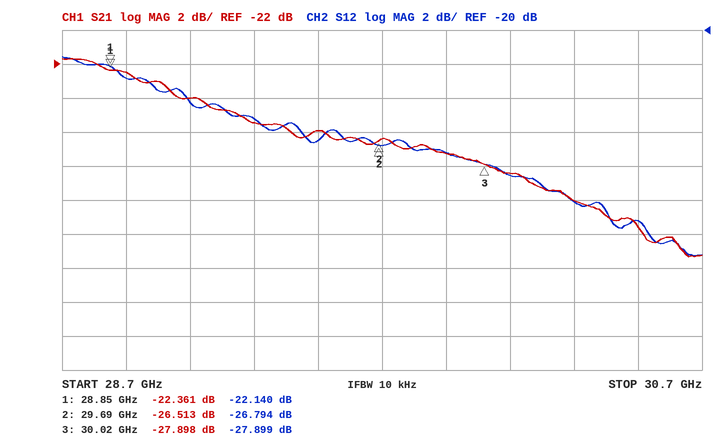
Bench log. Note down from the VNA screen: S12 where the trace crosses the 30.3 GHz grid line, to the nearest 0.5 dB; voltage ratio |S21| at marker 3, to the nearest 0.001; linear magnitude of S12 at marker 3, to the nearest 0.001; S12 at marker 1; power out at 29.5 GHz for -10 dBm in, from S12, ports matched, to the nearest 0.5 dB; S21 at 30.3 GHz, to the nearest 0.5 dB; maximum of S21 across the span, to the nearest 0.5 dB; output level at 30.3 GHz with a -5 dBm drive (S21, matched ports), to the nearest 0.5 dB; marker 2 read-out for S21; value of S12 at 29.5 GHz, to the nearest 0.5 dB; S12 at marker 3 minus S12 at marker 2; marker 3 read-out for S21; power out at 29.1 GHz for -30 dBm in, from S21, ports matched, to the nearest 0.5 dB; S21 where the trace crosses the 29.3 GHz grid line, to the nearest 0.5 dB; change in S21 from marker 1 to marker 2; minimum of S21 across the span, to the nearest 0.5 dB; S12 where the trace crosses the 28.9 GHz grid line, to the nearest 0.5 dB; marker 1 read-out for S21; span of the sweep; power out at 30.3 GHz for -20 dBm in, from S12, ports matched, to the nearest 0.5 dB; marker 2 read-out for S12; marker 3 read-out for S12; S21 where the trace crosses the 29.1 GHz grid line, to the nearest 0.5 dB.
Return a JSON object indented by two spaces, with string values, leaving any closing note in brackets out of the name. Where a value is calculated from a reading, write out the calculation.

{
  "S12 where the trace crosses the 30.3 GHz grid line, to the nearest 0.5 dB": "-30.0 dB",
  "voltage ratio |S21| at marker 3, to the nearest 0.001": "10^(-27.898/20) ≈ 0.040",
  "linear magnitude of S12 at marker 3, to the nearest 0.001": "10^(-27.899/20) ≈ 0.040",
  "S12 at marker 1": "-22.140 dB",
  "power out at 29.5 GHz for -10 dBm in, from S12, ports matched, to the nearest 0.5 dB": "-10 dBm + (-26.5 dB) = -36.5 dBm",
  "S21 at 30.3 GHz, to the nearest 0.5 dB": "-30.0 dB",
  "maximum of S21 across the span, to the nearest 0.5 dB": "-21.5 dB",
  "output level at 30.3 GHz with a -5 dBm drive (S21, matched ports), to the nearest 0.5 dB": "-5 dBm + (-30.0 dB) = -35.0 dBm",
  "marker 2 read-out for S21": "-26.513 dB",
  "value of S12 at 29.5 GHz, to the nearest 0.5 dB": "-26.5 dB",
  "S12 at marker 3 minus S12 at marker 2": "-27.899 − (-26.794) = -1.105 dB",
  "marker 3 read-out for S21": "-27.898 dB",
  "power out at 29.1 GHz for -30 dBm in, from S21, ports matched, to the nearest 0.5 dB": "-30 dBm + (-24.0 dB) = -54.0 dBm",
  "S21 where the trace crosses the 29.3 GHz grid line, to the nearest 0.5 dB": "-25.5 dB",
  "change in S21 from marker 1 to marker 2": "-26.513 − (-22.361) = -4.152 dB",
  "minimum of S21 across the span, to the nearest 0.5 dB": "-33.5 dB",
  "S12 where the trace crosses the 28.9 GHz grid line, to the nearest 0.5 dB": "-23.0 dB",
  "marker 1 read-out for S21": "-22.361 dB",
  "span of the sweep": "2 GHz",
  "power out at 30.3 GHz for -20 dBm in, from S12, ports matched, to the nearest 0.5 dB": "-20 dBm + (-30.0 dB) = -50.0 dBm",
  "marker 2 read-out for S12": "-26.794 dB",
  "marker 3 read-out for S12": "-27.899 dB",
  "S21 where the trace crosses the 29.1 GHz grid line, to the nearest 0.5 dB": "-24.0 dB"
}
